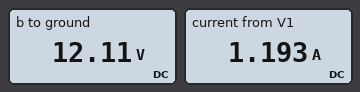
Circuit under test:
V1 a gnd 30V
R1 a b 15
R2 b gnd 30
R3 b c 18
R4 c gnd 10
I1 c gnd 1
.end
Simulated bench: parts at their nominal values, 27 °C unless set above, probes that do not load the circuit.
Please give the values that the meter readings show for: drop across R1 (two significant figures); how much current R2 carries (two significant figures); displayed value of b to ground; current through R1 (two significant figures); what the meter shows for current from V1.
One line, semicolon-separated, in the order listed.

18 V; 400 mA; 12.11 V; 1.2 A; 1.193 A
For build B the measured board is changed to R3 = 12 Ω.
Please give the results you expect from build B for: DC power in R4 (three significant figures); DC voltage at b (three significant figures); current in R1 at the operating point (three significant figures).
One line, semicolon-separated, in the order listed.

39.1 mW; 10.6 V; 1.29 A
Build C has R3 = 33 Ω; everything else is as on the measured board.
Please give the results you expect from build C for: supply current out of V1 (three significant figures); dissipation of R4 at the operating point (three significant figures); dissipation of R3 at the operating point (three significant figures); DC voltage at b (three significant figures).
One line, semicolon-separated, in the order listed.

1.04 A; 1.88 W; 10.6 W; 14.3 V
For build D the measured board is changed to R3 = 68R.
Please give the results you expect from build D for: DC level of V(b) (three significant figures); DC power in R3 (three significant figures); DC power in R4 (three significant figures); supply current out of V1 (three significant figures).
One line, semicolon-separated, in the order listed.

16.6 V; 7.90 W; 4.34 W; 894 mA
